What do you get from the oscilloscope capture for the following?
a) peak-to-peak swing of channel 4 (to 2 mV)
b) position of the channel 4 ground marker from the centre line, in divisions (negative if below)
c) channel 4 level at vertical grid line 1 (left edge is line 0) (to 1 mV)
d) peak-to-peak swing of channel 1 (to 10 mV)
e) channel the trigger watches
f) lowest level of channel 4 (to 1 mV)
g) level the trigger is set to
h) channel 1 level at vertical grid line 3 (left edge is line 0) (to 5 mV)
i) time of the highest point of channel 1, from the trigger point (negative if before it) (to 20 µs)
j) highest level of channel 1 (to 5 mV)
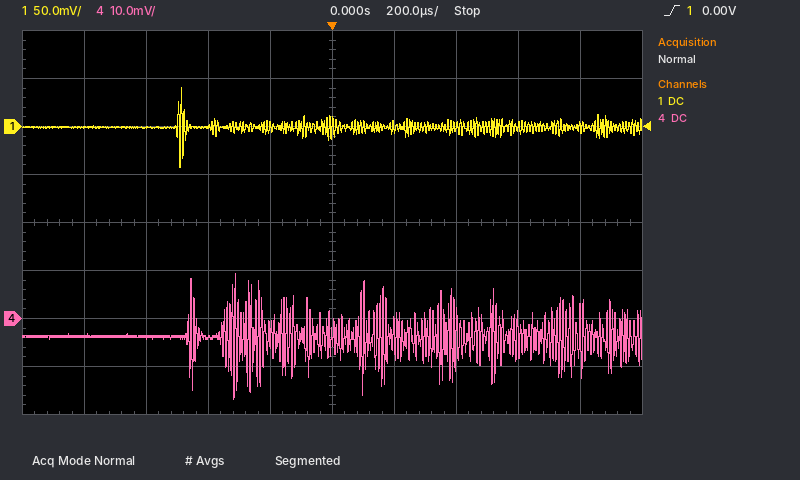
26 mV
-2.0 div
-4 mV
80 mV
channel 1
-17 mV
0.00 V
0 mV
-480 µs
40 mV
